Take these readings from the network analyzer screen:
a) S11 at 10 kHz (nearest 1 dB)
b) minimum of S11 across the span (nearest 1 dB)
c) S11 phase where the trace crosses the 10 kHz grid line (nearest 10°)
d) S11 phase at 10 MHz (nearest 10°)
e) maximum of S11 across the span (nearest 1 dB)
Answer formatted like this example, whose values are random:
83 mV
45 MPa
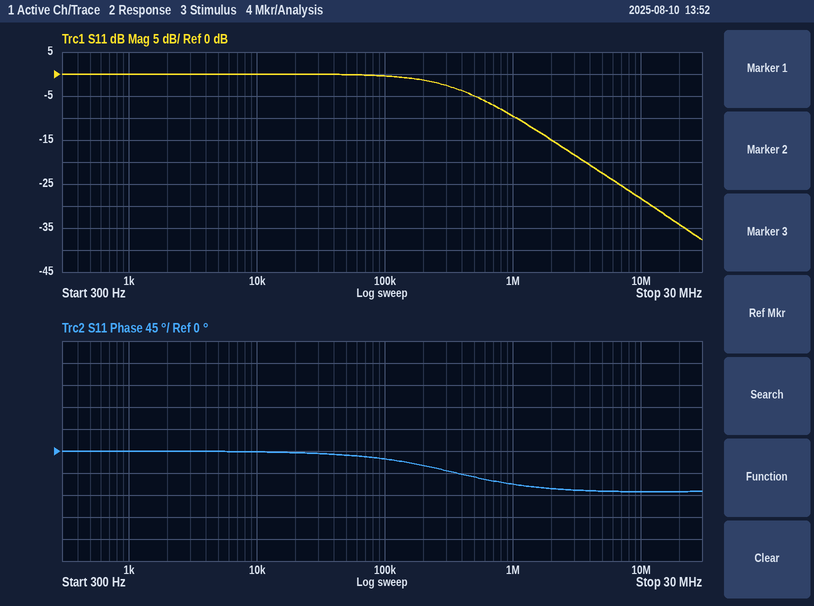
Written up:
0 dB
-38 dB
0°
-80°
0 dB
